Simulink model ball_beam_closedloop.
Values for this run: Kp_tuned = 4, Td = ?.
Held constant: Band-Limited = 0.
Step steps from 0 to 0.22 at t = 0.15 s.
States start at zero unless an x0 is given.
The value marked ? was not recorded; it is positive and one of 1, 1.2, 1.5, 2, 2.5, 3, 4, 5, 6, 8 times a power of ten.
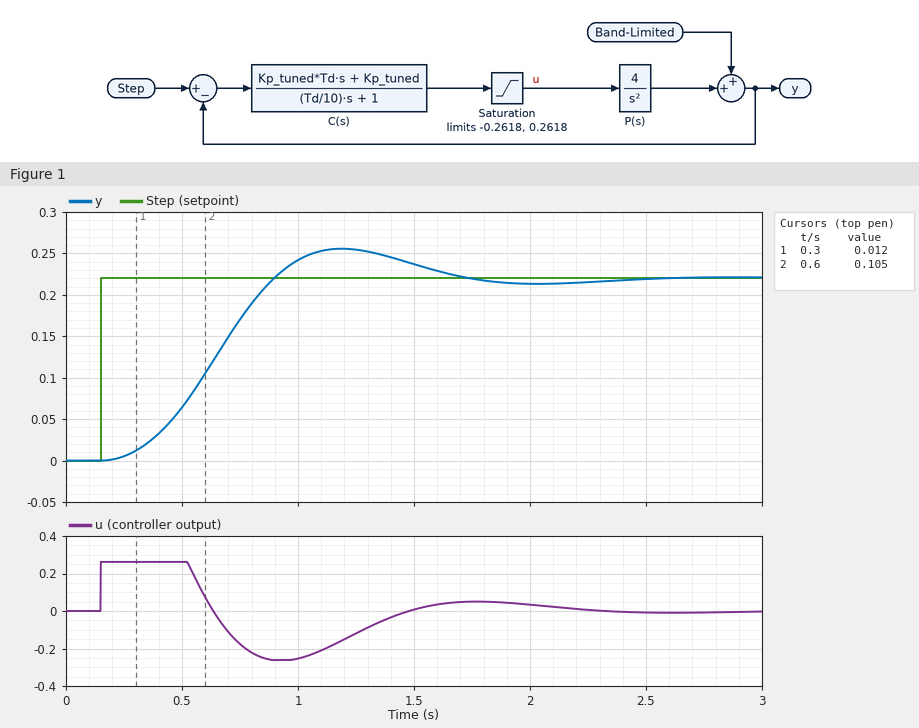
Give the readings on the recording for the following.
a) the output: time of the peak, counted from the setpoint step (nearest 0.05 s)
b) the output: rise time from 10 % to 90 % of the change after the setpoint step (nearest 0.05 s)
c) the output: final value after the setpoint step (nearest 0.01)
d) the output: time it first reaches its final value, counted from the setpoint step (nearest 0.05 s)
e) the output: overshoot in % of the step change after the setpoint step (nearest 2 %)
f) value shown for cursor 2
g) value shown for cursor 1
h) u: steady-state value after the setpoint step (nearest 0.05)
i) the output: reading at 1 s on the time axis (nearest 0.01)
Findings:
1.05 s
0.45 s
0.22
0.75 s
16 %
0.105
0.012
0.00
0.24
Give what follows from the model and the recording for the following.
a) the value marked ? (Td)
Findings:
0.25
